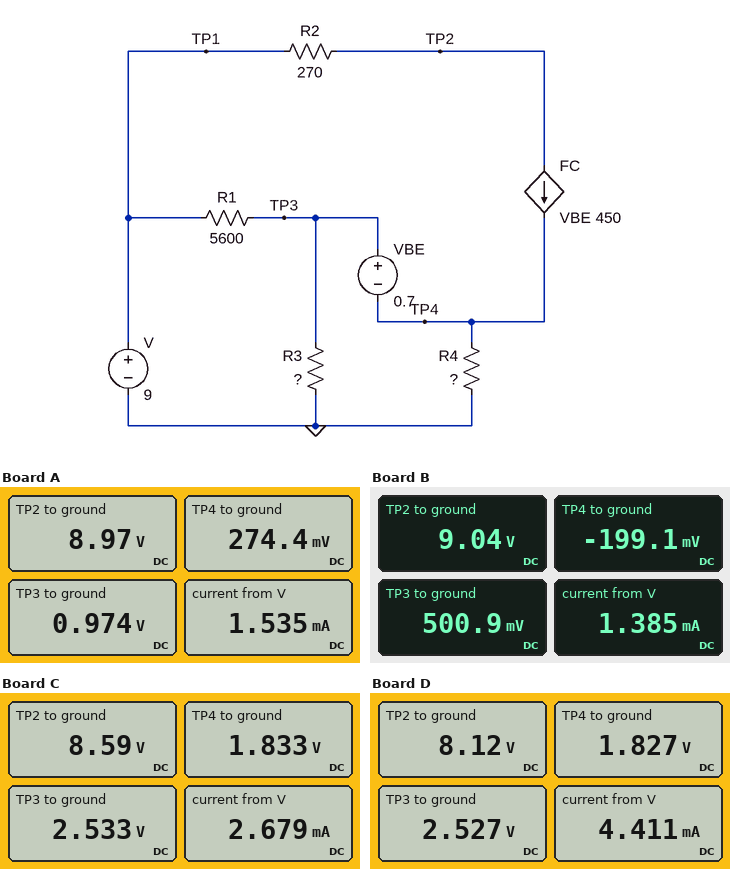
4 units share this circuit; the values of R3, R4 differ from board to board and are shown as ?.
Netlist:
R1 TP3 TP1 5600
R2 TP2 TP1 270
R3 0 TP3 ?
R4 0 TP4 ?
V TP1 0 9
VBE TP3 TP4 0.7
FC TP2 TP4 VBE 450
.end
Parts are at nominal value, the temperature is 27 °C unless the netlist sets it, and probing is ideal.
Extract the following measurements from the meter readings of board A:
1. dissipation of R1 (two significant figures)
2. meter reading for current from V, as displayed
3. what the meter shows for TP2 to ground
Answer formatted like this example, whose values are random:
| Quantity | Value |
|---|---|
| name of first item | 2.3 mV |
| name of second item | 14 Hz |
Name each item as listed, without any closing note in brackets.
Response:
| Quantity | Value |
|---|---|
| dissipation of R1 | 12 mW |
| meter reading for current from V, as displayed | 1.535 mA |
| what the meter shows for TP2 to ground | 8.97 V |
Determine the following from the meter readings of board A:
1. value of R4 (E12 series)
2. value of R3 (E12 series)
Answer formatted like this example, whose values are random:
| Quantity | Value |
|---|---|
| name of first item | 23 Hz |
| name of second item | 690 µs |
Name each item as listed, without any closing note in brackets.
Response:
| Quantity | Value |
|---|---|
| value of R4 | 2.7 kΩ |
| value of R3 | 680 Ω |
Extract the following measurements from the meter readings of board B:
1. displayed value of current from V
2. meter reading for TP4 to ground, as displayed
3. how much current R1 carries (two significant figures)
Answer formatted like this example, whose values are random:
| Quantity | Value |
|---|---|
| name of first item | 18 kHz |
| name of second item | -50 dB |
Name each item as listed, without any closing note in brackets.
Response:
| Quantity | Value |
|---|---|
| displayed value of current from V | 1.385 mA |
| meter reading for TP4 to ground, as displayed | -199.1 mV |
| how much current R1 carries | 1.5 mA |
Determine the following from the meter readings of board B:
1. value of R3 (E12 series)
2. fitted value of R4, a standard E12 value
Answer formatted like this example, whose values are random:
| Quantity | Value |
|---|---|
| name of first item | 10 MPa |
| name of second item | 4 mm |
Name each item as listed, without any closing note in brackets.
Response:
| Quantity | Value |
|---|---|
| value of R3 | 330 Ω |
| fitted value of R4, a standard E12 value | 1.5 kΩ |
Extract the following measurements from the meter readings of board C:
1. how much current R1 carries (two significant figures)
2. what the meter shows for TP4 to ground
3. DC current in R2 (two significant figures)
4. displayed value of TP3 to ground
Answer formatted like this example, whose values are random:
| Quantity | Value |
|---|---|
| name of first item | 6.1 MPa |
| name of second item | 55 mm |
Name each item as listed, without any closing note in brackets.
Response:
| Quantity | Value |
|---|---|
| how much current R1 carries | 1.2 mA |
| what the meter shows for TP4 to ground | 1.833 V |
| DC current in R2 | 1.5 mA |
| displayed value of TP3 to ground | 2.533 V |
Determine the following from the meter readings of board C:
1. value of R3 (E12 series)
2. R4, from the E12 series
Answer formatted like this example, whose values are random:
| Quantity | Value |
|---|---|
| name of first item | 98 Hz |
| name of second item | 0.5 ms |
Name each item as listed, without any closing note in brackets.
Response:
| Quantity | Value |
|---|---|
| value of R3 | 2.2 kΩ |
| R4, from the E12 series | 1.2 kΩ |
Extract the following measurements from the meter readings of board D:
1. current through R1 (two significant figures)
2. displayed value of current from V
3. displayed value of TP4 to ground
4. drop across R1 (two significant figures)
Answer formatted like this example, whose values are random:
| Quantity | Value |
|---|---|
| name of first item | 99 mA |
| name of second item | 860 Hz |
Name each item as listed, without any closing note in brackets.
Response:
| Quantity | Value |
|---|---|
| current through R1 | 1.2 mA |
| displayed value of current from V | 4.411 mA |
| displayed value of TP4 to ground | 1.827 V |
| drop across R1 | 6.5 V |
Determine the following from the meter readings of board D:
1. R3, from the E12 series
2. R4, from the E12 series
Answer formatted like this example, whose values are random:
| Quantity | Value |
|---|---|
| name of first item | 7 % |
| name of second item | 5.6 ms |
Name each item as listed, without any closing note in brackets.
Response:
| Quantity | Value |
|---|---|
| R3, from the E12 series | 2.2 kΩ |
| R4, from the E12 series | 560 Ω |
